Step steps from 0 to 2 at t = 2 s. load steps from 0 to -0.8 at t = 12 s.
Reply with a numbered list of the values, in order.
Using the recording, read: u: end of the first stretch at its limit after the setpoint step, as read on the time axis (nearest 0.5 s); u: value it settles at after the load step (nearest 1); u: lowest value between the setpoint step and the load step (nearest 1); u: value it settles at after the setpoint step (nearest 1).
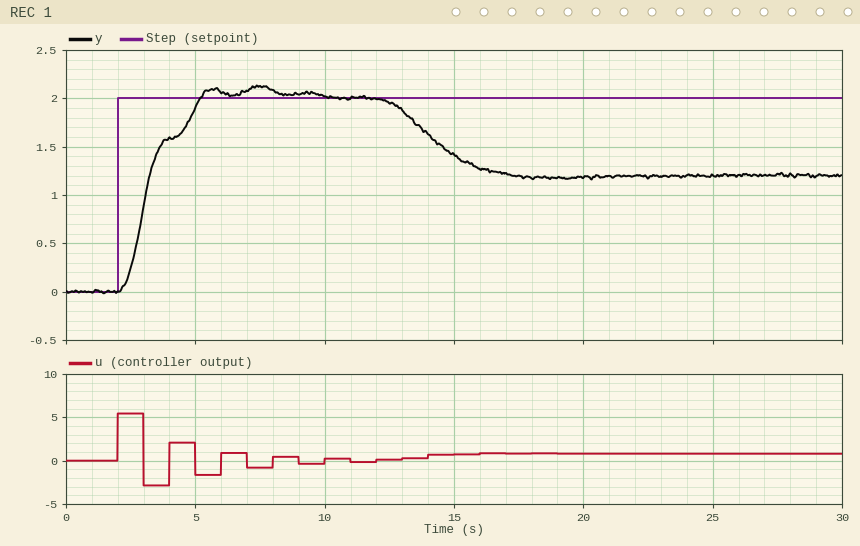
1. 3.0 s
2. 1
3. -3
4. 0
